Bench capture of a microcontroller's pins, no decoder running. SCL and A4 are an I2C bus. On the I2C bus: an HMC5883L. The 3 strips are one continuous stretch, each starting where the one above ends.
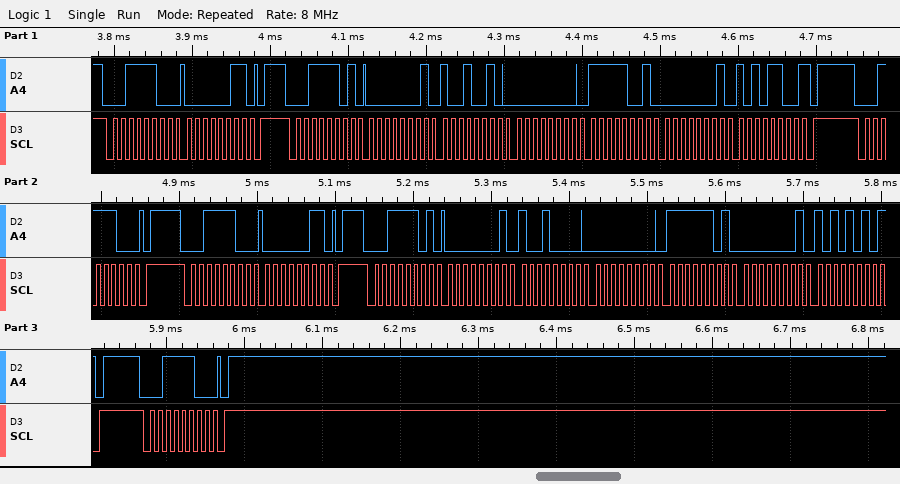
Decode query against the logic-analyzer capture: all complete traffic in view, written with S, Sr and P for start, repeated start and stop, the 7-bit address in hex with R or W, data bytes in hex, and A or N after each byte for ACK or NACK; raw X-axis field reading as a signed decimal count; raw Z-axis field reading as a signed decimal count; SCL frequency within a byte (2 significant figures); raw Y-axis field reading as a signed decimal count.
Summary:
S 1EW A 03 A P S 1ER A 01 A 92 A 00 A F9 A 01 A AC N P S 1EW A P S 1EW A 03 A P S 1ER A 01 A 90 A 00 A FD A 01 A AA N P S 1EW A P
402
249
100 kHz
428
